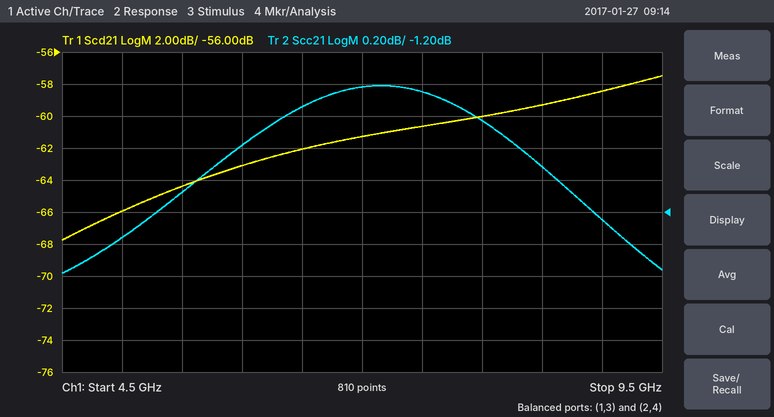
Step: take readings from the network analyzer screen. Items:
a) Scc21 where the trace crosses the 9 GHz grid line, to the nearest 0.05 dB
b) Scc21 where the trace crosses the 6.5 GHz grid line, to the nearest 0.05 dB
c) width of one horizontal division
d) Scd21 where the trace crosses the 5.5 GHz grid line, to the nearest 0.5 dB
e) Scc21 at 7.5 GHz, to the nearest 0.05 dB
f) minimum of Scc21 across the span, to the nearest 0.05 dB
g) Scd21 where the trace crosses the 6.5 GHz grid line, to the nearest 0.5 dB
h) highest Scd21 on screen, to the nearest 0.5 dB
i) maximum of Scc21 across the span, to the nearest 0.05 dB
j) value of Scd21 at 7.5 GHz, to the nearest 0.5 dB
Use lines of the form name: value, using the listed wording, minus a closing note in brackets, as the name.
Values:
Scc21 where the trace crosses the 9 GHz grid line, to the nearest 0.05 dB: -1.25 dB
Scc21 where the trace crosses the 6.5 GHz grid line, to the nearest 0.05 dB: -0.55 dB
width of one horizontal division: 500 MHz
Scd21 where the trace crosses the 5.5 GHz grid line, to the nearest 0.5 dB: -64.5 dB
Scc21 at 7.5 GHz, to the nearest 0.05 dB: -0.45 dB
minimum of Scc21 across the span, to the nearest 0.05 dB: -1.60 dB
Scd21 where the trace crosses the 6.5 GHz grid line, to the nearest 0.5 dB: -62.0 dB
highest Scd21 on screen, to the nearest 0.5 dB: -57.5 dB
maximum of Scc21 across the span, to the nearest 0.05 dB: -0.40 dB
value of Scd21 at 7.5 GHz, to the nearest 0.5 dB: -60.5 dB
